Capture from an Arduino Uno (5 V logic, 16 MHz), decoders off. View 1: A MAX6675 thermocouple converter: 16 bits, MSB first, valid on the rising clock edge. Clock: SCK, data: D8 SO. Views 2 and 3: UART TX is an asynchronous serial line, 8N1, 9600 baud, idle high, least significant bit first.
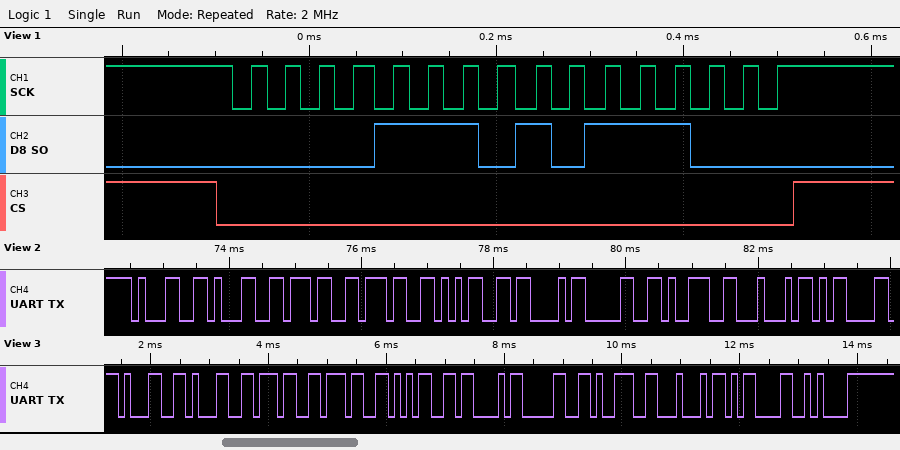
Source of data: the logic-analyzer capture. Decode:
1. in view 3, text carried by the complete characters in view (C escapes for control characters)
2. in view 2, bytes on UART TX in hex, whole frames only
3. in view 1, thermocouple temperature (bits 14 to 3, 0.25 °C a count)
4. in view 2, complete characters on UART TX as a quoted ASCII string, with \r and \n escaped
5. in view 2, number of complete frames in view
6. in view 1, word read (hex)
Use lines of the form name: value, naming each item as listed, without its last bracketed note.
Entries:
in view 3, text carried by the complete characters in view: "11775C09D\r\n"
in view 2, bytes on UART TX in hex, whole frames only: 0x31 0x31 0x37 0x37 0x35 0x43 0x30 0x39 0x44 0x0D
in view 1, thermocouple temperature: 117.75 °C
in view 2, complete characters on UART TX as a quoted ASCII string, with \r and \n escaped: "11775C09D\r"
in view 2, number of complete frames in view: 10
in view 1, word read: 0x0EB8
